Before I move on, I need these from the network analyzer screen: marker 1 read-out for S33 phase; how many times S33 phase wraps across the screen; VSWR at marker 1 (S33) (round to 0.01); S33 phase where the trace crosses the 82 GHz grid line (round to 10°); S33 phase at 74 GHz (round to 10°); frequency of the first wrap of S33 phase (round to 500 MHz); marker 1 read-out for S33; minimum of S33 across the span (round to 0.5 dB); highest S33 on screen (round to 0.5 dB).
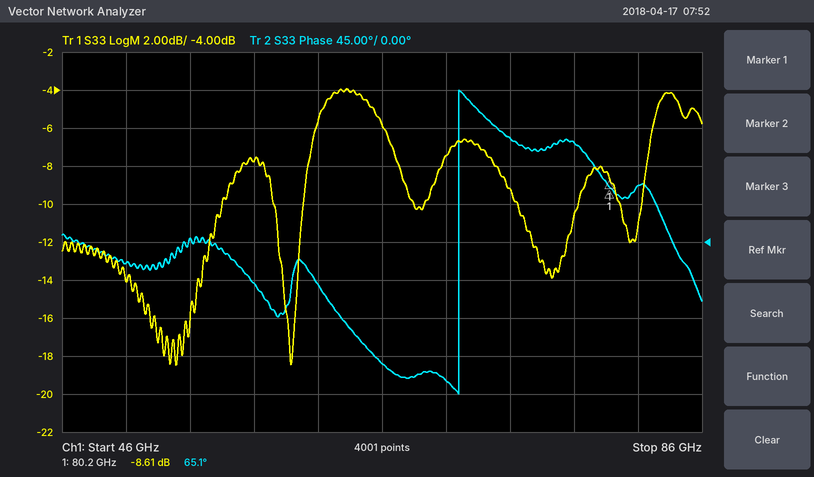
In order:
65.1°
1
2.18
70°
120°
71.0 GHz
-8.61 dB
-18.5 dB
-4.0 dB
